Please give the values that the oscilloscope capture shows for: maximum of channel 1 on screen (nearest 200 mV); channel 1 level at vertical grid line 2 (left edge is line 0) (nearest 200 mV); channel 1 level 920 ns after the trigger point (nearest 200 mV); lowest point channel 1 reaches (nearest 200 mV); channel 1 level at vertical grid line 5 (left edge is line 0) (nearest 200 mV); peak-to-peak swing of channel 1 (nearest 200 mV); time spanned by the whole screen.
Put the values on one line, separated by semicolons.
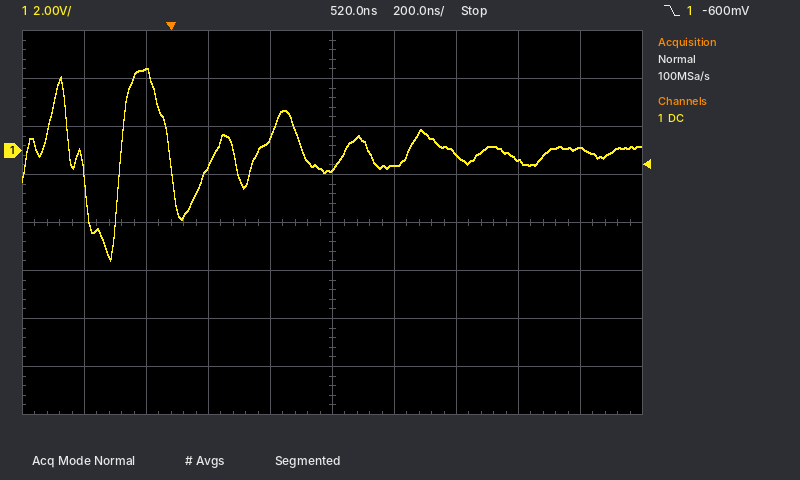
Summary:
3.4 V; 3.4 V; -200 mV; -4.6 V; -800 mV; 8.0 V; 2 µs
